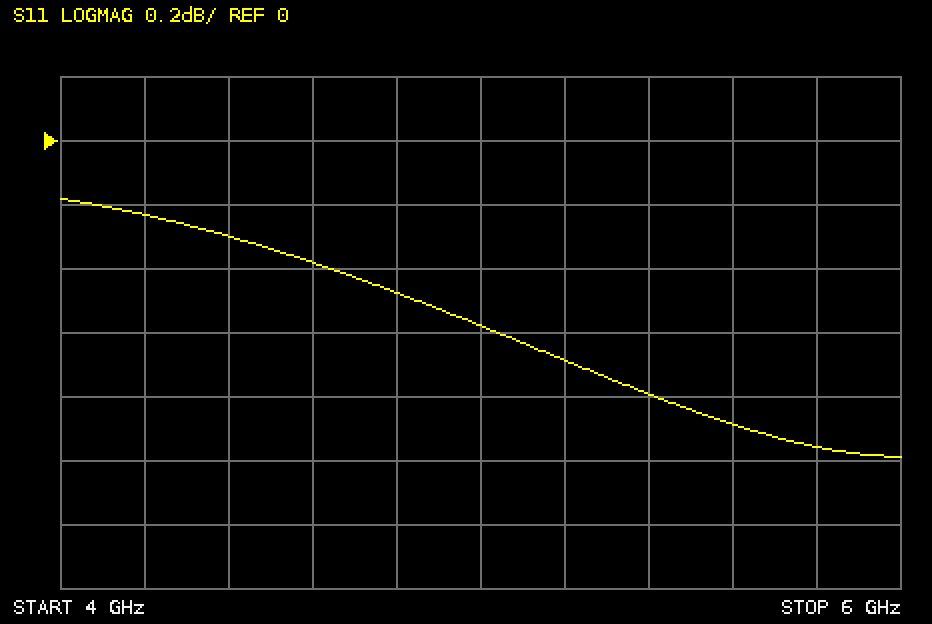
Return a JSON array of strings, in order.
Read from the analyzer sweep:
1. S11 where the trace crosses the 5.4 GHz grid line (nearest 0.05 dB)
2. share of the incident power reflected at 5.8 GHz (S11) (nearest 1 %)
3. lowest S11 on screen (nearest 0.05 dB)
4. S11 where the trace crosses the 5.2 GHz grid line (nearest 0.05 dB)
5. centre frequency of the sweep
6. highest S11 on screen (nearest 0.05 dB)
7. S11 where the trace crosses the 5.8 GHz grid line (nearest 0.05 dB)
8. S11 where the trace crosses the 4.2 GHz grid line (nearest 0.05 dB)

["-0.80 dB", "80 %", "-1.00 dB", "-0.70 dB", "5 GHz", "-0.20 dB", "-0.95 dB", "-0.25 dB"]
